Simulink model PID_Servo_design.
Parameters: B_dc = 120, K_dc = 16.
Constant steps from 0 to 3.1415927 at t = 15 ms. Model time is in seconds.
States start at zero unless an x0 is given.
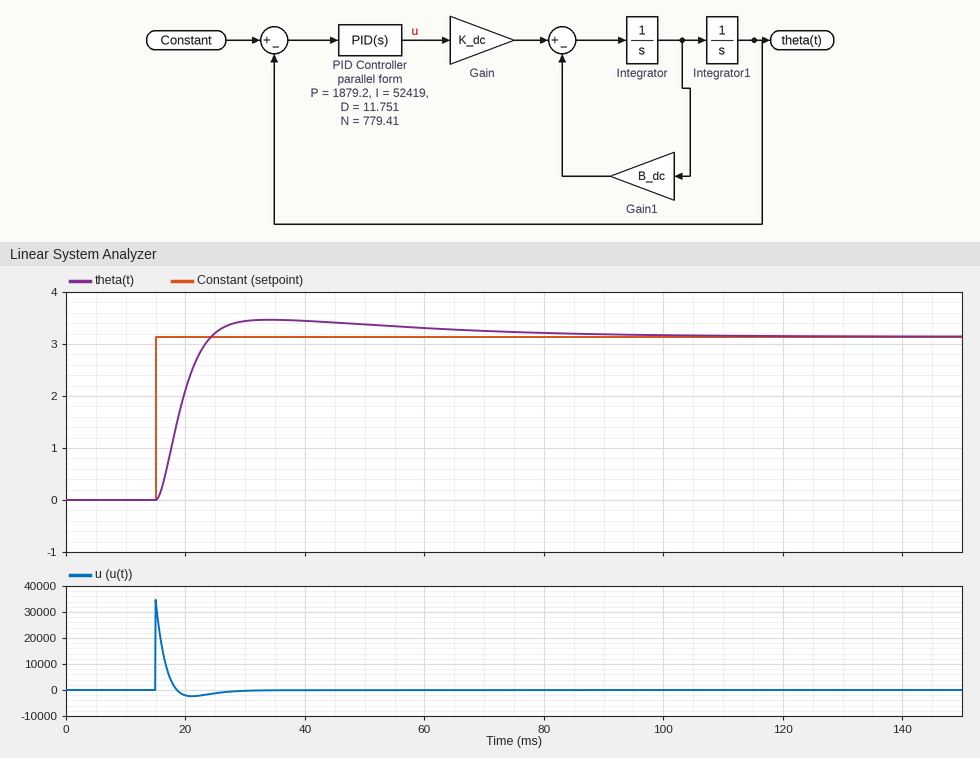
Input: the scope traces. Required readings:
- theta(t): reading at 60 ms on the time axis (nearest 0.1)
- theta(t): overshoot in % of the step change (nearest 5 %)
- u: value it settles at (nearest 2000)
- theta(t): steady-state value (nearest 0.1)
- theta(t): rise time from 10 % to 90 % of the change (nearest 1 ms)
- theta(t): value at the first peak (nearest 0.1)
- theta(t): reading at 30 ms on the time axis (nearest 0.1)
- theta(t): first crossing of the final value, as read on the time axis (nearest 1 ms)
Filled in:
3.3
10 %
0
3.1
6 ms
3.5
3.4
24 ms
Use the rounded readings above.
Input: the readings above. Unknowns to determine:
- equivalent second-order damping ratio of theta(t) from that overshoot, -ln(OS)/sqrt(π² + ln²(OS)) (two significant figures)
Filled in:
0.59
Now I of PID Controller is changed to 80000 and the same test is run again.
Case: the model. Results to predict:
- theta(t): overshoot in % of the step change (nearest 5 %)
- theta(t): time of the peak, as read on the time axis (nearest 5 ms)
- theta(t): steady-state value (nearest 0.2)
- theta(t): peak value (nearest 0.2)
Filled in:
15 %
35 ms
3.2
3.6
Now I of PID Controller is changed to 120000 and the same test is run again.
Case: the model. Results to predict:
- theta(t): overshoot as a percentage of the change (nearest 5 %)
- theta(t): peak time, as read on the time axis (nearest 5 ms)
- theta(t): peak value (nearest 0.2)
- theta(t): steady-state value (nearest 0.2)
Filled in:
20 %
35 ms
3.8
3.2
